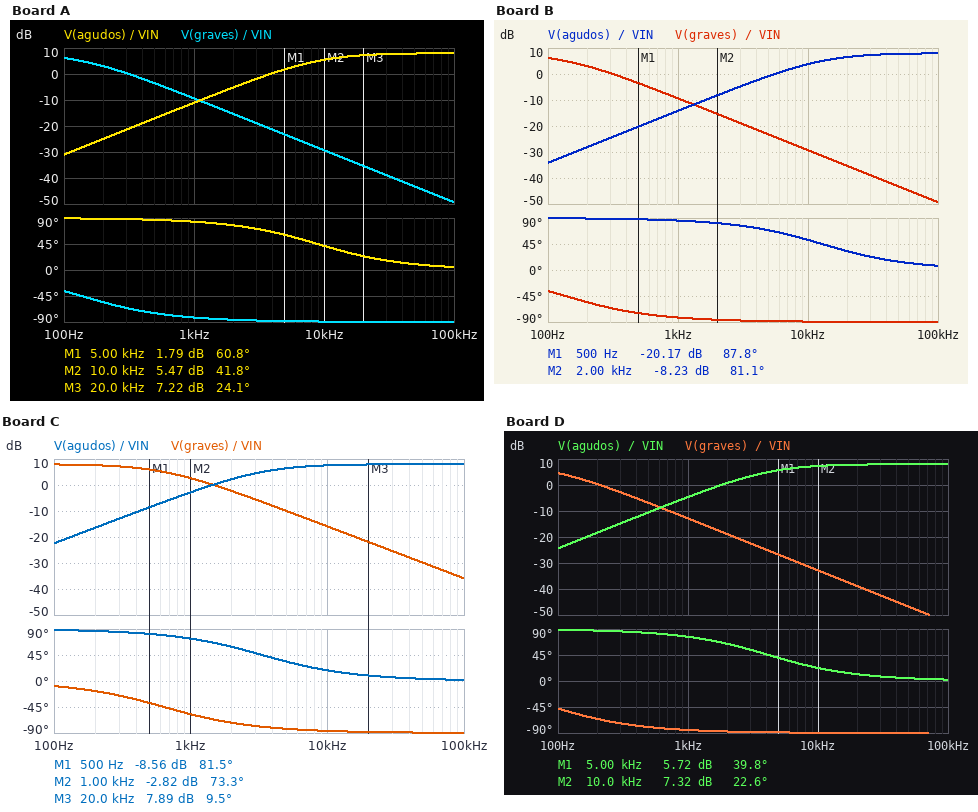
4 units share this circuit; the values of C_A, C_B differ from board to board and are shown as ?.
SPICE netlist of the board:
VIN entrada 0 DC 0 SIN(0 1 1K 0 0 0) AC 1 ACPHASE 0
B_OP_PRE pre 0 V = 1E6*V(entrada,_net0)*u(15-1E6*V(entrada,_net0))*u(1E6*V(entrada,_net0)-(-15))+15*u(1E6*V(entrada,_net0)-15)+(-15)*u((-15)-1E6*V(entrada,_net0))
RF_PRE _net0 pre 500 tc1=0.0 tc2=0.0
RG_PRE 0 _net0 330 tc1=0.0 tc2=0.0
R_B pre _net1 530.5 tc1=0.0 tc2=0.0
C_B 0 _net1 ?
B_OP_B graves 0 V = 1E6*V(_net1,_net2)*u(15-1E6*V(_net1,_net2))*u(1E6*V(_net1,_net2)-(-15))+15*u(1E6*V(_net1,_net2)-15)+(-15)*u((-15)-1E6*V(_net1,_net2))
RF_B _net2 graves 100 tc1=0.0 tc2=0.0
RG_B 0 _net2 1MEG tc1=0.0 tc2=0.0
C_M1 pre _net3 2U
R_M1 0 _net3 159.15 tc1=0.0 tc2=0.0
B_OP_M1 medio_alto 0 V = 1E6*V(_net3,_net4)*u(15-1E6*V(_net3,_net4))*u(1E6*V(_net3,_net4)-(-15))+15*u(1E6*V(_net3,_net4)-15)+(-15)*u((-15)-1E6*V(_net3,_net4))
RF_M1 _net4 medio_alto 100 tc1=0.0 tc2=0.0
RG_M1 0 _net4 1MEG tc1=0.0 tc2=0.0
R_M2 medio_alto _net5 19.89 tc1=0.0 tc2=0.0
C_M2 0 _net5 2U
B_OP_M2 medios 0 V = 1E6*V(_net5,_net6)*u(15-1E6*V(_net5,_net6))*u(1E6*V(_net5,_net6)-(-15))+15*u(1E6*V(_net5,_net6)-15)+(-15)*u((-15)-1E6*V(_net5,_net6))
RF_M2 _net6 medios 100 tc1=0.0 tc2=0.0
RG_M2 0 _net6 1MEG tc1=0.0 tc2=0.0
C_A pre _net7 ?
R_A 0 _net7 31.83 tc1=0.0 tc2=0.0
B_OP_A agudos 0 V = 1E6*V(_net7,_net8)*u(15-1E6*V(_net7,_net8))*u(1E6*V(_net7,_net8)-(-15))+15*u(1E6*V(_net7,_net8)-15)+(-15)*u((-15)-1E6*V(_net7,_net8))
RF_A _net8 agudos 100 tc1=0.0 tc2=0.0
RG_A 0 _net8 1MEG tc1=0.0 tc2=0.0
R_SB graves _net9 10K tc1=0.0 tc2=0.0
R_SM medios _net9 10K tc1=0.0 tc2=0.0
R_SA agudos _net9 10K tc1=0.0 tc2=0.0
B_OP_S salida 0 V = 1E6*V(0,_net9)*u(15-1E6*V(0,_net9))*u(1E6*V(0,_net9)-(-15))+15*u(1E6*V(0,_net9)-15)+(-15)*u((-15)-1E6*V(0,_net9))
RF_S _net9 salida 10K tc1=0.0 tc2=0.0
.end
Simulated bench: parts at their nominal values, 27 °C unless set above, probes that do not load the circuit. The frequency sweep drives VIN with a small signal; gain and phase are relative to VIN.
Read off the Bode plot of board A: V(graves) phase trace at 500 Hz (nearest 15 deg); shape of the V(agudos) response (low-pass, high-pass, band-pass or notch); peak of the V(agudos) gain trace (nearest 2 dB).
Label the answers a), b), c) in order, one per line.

a) -75 deg
b) high-pass
c) 8 dB
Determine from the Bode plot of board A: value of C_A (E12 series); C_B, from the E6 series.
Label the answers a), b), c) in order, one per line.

a) 560 nF
b) 2.2 µF
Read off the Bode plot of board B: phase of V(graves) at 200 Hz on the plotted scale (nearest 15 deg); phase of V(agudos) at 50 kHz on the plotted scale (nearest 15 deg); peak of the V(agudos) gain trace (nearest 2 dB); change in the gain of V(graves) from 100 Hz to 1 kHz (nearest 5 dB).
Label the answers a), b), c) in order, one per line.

a) -60 deg
b) 15 deg
c) 8 dB
d) -15 dB
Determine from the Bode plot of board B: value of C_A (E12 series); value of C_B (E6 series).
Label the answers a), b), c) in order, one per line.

a) 390 nF
b) 2.2 µF
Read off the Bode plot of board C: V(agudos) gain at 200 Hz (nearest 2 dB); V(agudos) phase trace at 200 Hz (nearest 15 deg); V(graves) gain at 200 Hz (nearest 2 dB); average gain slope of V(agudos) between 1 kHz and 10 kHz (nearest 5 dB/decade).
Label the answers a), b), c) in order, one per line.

a) -16 dB
b) 90 deg
c) 8 dB
d) 10 dB/decade
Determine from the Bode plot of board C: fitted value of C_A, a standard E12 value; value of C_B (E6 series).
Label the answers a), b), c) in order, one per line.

a) 1.5 µF
b) 470 nF
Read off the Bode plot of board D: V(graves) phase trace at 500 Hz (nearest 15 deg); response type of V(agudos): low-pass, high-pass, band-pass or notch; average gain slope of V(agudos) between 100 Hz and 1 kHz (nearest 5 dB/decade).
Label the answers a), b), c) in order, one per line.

a) -75 deg
b) high-pass
c) 20 dB/decade
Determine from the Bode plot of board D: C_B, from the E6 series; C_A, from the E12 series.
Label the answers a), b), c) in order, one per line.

a) 3.3 µF
b) 1.2 µF
